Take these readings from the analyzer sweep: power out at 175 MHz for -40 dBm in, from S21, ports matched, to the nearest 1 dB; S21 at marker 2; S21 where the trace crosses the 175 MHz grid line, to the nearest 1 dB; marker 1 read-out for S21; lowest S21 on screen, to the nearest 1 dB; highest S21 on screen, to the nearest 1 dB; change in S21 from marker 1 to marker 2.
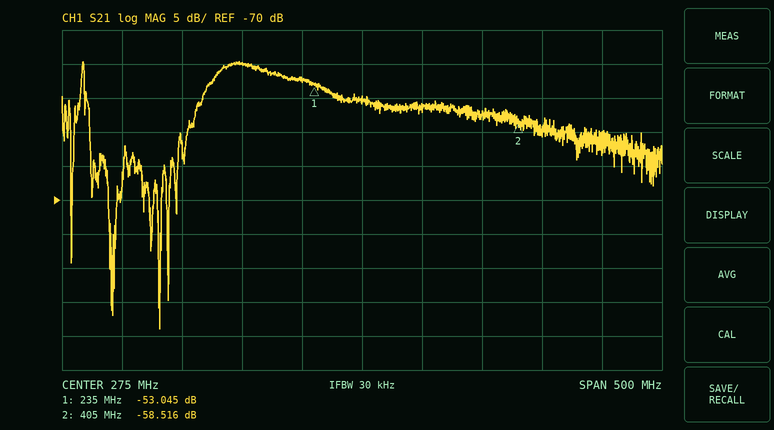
-90 dBm
-58.516 dB
-50 dB
-53.045 dB
-89 dB
-50 dB
-5.471 dB
